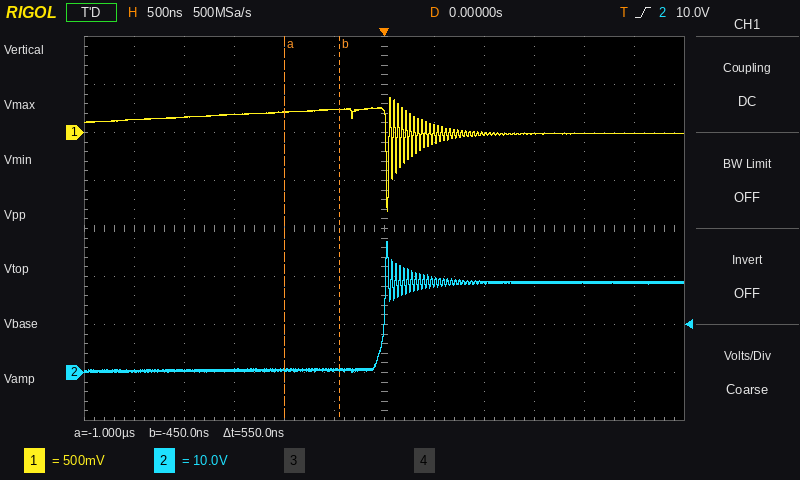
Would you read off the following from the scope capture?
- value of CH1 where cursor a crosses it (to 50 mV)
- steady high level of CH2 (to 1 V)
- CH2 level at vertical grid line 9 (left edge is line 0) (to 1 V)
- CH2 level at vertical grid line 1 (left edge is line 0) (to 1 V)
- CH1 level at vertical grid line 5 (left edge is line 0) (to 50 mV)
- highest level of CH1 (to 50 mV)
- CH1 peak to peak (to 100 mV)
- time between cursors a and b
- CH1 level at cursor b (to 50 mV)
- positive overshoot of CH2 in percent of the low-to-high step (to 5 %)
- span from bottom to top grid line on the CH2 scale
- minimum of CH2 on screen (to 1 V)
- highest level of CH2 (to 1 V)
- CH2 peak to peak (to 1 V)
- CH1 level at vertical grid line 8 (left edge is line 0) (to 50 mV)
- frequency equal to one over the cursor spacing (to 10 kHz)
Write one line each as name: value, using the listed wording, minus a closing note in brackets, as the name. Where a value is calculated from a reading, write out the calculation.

value of CH1 where cursor a crosses it: 200 mV
steady high level of CH2: 19 V
CH2 level at vertical grid line 9 (left edge is line 0): 19 V
CH2 level at vertical grid line 1 (left edge is line 0): 0 V
CH1 level at vertical grid line 5 (left edge is line 0): 250 mV
highest level of CH1: 350 mV
CH1 peak to peak: 1.20 V
time between cursors a and b: 550 ns
CH1 level at cursor b: 250 mV
positive overshoot of CH2 in percent of the low-to-high step: 45 %
span from bottom to top grid line on the CH2 scale: 80 V
minimum of CH2 on screen: 0 V
highest level of CH2: 27 V
CH2 peak to peak: 27 V − (0 V) = 27 V
CH1 level at vertical grid line 8 (left edge is line 0): 0 mV
frequency equal to one over the cursor spacing: 1 / 550 ns ≈ 1.82 MHz
